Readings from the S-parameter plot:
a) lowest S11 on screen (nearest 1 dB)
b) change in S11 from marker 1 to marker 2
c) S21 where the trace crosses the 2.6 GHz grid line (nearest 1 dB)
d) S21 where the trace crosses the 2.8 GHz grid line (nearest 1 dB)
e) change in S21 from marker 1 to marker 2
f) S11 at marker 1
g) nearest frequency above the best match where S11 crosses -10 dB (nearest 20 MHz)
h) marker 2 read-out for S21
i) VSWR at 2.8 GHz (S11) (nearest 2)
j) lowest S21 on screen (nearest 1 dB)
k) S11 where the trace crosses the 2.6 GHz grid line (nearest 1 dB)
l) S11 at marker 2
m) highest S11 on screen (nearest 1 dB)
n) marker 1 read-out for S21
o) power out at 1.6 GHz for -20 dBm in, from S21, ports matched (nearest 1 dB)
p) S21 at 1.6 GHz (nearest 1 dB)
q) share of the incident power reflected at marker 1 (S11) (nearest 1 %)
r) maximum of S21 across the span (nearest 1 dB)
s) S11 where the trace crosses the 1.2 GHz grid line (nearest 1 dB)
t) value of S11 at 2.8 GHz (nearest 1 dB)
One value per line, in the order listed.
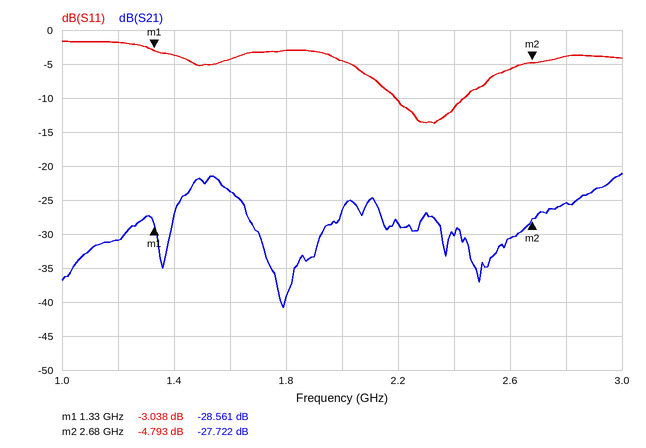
-14 dB
-1.755 dB
-31 dB
-25 dB
0.839 dB
-3.038 dB
2.44 GHz
-27.722 dB
4
-41 dB
-6 dB
-4.793 dB
-2 dB
-28.561 dB
-44 dBm
-24 dB
50 %
-21 dB
-2 dB
-4 dB
